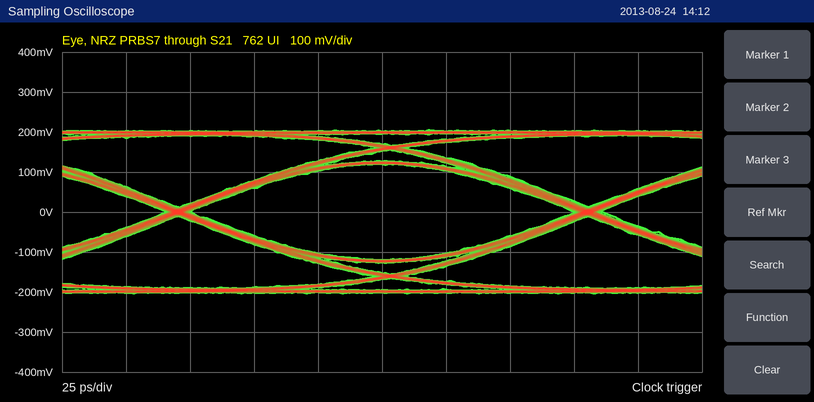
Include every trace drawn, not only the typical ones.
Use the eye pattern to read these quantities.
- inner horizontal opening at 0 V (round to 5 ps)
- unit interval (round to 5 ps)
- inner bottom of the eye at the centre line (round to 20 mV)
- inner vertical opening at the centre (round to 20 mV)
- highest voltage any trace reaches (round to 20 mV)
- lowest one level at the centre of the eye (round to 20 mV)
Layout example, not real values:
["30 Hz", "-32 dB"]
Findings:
["150 ps", "160 ps", "-120 mV", "240 mV", "200 mV", "120 mV"]
